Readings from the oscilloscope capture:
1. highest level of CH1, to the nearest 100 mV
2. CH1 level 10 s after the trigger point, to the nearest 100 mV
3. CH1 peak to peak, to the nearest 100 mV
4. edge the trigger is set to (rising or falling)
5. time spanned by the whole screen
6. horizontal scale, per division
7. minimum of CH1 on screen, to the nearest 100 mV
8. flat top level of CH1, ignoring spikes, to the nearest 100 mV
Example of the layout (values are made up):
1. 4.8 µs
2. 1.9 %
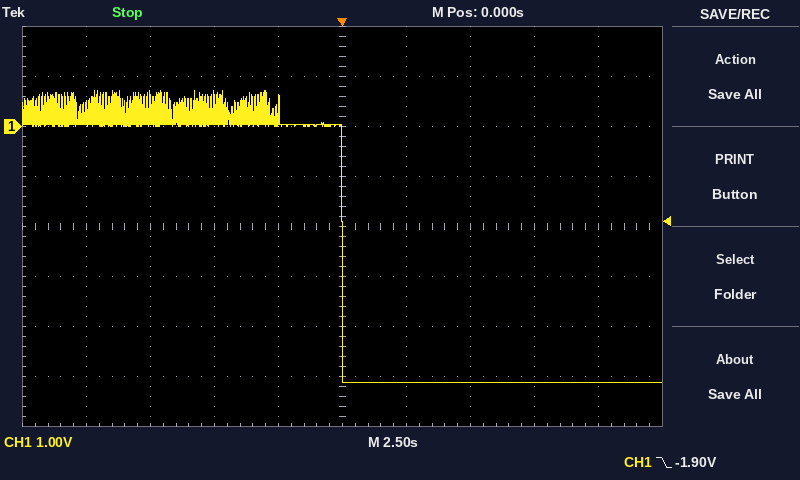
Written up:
1. 700 mV
2. -5.1 V
3. 5.8 V
4. falling
5. 25 s
6. 2.5 s
7. -5.1 V
8. 0.0 V
